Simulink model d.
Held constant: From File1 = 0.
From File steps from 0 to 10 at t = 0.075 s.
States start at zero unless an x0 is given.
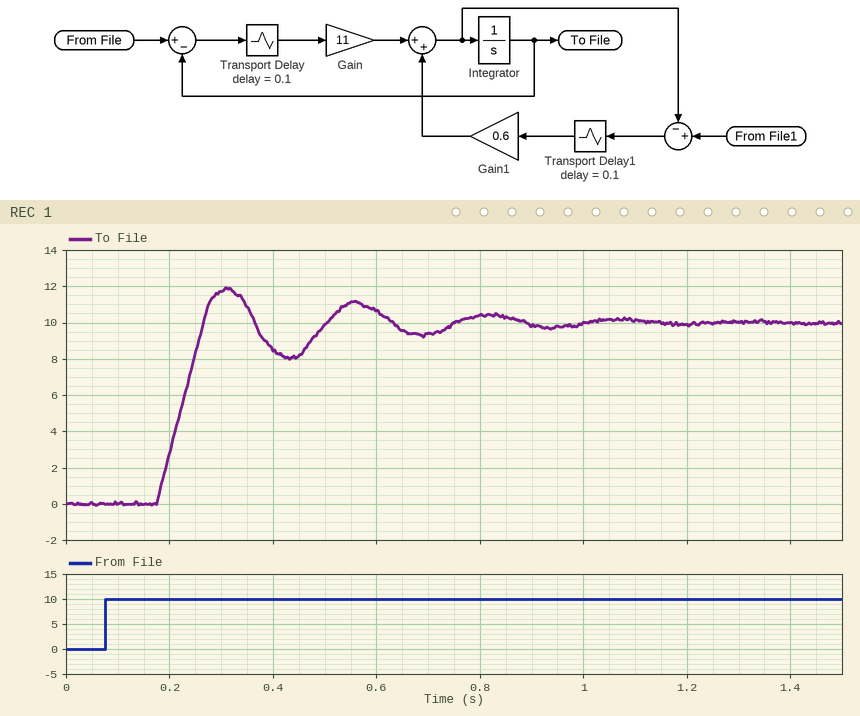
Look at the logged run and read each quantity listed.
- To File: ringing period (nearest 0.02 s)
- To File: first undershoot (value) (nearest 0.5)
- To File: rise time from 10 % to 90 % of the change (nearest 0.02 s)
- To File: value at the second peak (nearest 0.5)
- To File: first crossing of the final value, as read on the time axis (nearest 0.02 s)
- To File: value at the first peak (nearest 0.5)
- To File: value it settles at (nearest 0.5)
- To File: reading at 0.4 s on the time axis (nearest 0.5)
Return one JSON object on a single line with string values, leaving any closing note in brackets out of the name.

{"To File: ringing period": "0.24 s", "To File: first undershoot (value)": "8.0", "To File: rise time from 10 % to 90 % of the change": "0.08 s", "To File: value at the second peak": "11.0", "To File: first crossing of the final value, as read on the time axis": "0.26 s", "To File: value at the first peak": "12.0", "To File: value it settles at": "10.0", "To File: reading at 0.4 s on the time axis": "8.5"}
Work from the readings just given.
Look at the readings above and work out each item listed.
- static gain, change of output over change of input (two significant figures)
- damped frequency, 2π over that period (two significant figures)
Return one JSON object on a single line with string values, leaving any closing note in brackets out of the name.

{"static gain, change of output over change of input": "1.0", "damped frequency, 2π over that period": "26 rad/s"}
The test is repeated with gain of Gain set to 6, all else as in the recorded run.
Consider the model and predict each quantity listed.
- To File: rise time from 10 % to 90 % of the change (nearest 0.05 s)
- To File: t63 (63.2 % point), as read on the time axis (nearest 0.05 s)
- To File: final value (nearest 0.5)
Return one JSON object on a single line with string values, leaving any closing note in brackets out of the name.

{"To File: rise time from 10 % to 90 % of the change": "0.45 s", "To File: t63 (63.2 % point), as read on the time axis": "0.30 s", "To File: final value": "10.0"}
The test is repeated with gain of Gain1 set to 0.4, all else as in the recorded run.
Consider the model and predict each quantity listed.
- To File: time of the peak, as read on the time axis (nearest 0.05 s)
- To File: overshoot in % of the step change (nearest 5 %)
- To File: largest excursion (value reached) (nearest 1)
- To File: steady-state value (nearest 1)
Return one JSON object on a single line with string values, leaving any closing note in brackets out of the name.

{"To File: time of the peak, as read on the time axis": "0.35 s", "To File: overshoot in % of the step change": "30 %", "To File: largest excursion (value reached)": "13", "To File: steady-state value": "10"}
